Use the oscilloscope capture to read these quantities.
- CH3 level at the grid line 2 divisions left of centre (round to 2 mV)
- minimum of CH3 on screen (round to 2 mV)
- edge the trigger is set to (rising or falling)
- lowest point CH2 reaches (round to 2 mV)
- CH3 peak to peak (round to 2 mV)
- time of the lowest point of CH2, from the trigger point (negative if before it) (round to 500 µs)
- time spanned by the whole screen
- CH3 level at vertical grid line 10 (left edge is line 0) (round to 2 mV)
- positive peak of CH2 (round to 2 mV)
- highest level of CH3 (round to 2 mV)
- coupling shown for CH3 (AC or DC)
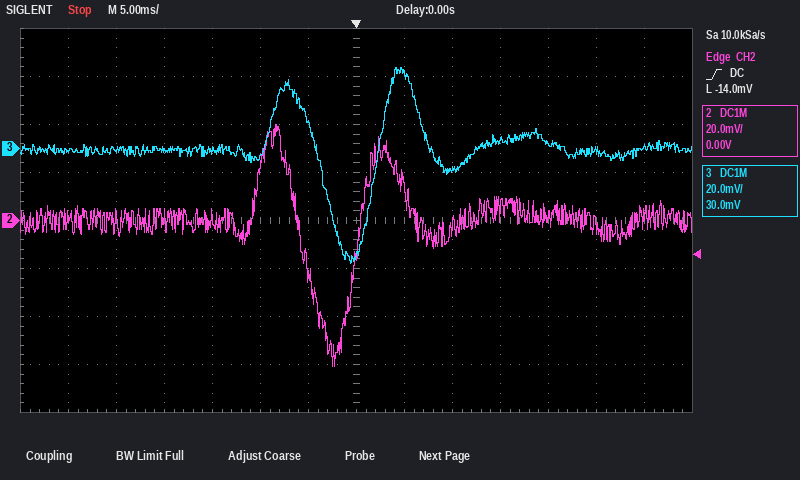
-4 mV
-48 mV
rising
-60 mV
82 mV
-2.5 ms
70 ms
4 mV
40 mV
34 mV
DC
